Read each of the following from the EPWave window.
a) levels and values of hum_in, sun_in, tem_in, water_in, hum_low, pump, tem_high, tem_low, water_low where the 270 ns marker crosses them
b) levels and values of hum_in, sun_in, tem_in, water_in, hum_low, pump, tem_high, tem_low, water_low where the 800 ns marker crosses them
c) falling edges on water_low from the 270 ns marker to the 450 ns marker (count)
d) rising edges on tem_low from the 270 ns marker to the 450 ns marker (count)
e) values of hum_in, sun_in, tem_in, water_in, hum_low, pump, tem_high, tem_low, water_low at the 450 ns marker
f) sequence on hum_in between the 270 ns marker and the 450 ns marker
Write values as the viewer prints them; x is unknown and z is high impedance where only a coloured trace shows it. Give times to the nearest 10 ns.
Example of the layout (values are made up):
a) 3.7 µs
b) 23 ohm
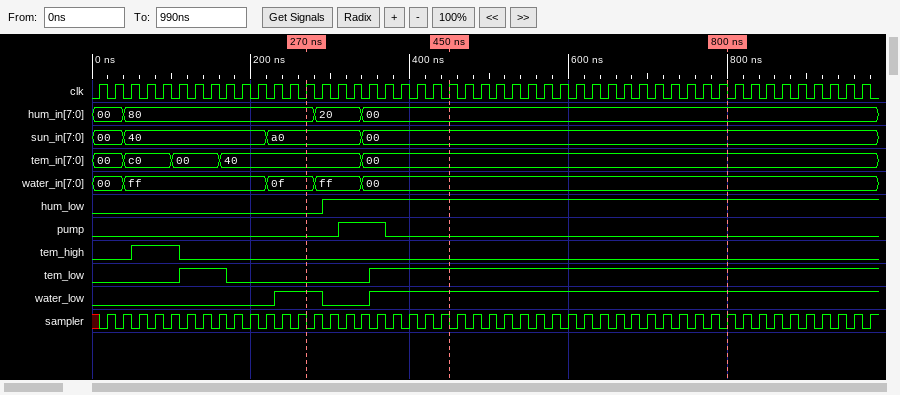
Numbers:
a) hum_in=80, sun_in=a0, tem_in=40, water_in=0f, hum_low=0, pump=0, tem_high=0, tem_low=0, water_low=1
b) hum_in=00, sun_in=00, tem_in=00, water_in=00, hum_low=1, pump=0, tem_high=0, tem_low=1, water_low=1
c) 1
d) 1
e) hum_in=00, sun_in=00, tem_in=00, water_in=00, hum_low=1, pump=0, tem_high=0, tem_low=1, water_low=1
f) 80, 20, 00
